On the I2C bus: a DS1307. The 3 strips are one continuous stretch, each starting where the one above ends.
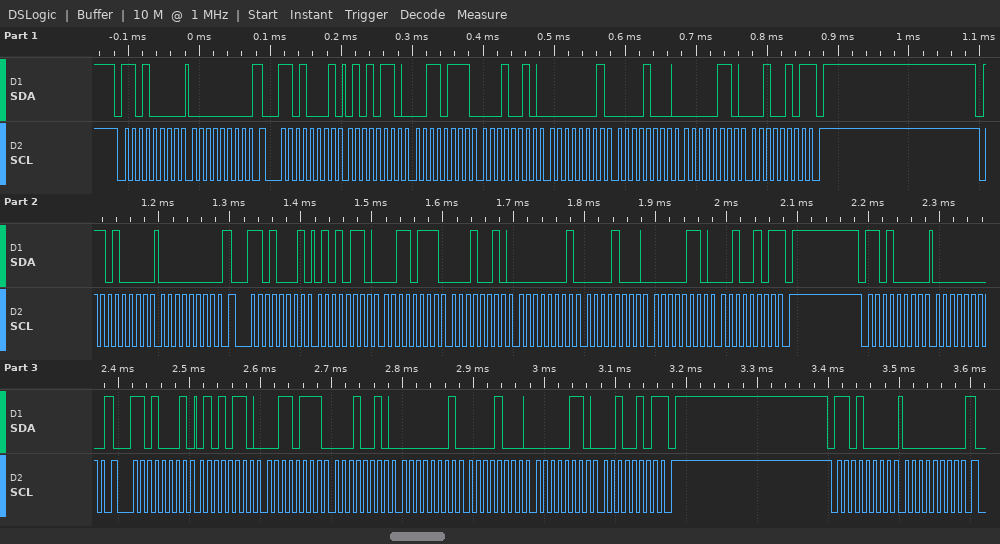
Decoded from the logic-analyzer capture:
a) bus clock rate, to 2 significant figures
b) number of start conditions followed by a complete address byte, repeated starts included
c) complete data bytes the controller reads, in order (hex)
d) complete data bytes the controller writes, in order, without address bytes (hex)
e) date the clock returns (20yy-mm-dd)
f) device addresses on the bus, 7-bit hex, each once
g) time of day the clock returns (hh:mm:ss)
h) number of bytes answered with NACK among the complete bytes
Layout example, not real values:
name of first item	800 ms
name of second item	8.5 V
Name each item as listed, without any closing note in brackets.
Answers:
bus clock rate, to 2 significant figures	100 kHz
number of start conditions followed by a complete address byte, repeated starts included	7
complete data bytes the controller reads, in order	56 37 12 01 08 06 25 56 37 12 01 08 06 25 56 37 12 01 08 06 25
complete data bytes the controller writes, in order, without address bytes	00 00 00 00
date the clock returns	2025-06-08
device addresses on the bus, 7-bit hex, each once	0x68
time of day the clock returns	12:37:56
number of bytes answered with NACK among the complete bytes	3
